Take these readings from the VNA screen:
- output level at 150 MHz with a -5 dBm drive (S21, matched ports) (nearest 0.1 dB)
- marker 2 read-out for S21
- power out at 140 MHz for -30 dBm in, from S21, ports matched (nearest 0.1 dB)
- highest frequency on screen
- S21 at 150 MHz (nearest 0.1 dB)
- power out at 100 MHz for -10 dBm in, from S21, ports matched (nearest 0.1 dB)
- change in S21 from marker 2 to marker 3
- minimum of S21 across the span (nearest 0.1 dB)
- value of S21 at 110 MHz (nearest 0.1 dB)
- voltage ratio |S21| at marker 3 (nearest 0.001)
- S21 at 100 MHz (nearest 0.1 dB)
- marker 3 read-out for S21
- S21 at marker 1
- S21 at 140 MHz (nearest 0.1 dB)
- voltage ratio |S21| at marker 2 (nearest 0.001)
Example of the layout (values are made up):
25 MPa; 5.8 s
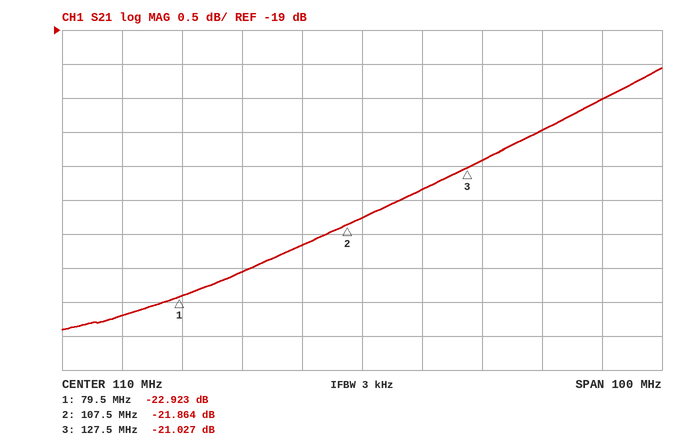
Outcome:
-25.0 dBm; -21.864 dB; -50.5 dBm; 160 MHz; -20.0 dB; -32.2 dBm; 0.837 dB; -23.4 dB; -21.8 dB; 0.089; -22.2 dB; -21.027 dB; -22.923 dB; -20.5 dB; 0.081
